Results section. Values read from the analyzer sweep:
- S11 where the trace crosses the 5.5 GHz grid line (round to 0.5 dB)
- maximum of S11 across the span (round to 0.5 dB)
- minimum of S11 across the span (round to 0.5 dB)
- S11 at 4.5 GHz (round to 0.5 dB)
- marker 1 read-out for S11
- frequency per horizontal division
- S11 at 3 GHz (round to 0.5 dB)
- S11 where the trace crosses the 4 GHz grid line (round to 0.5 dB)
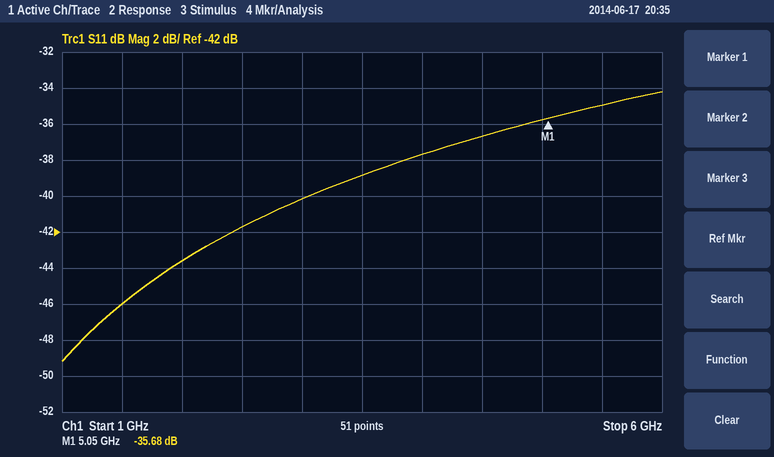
-35.0 dB
-34.0 dB
-49.0 dB
-36.5 dB
-35.68 dB
500 MHz
-40.0 dB
-37.5 dB
